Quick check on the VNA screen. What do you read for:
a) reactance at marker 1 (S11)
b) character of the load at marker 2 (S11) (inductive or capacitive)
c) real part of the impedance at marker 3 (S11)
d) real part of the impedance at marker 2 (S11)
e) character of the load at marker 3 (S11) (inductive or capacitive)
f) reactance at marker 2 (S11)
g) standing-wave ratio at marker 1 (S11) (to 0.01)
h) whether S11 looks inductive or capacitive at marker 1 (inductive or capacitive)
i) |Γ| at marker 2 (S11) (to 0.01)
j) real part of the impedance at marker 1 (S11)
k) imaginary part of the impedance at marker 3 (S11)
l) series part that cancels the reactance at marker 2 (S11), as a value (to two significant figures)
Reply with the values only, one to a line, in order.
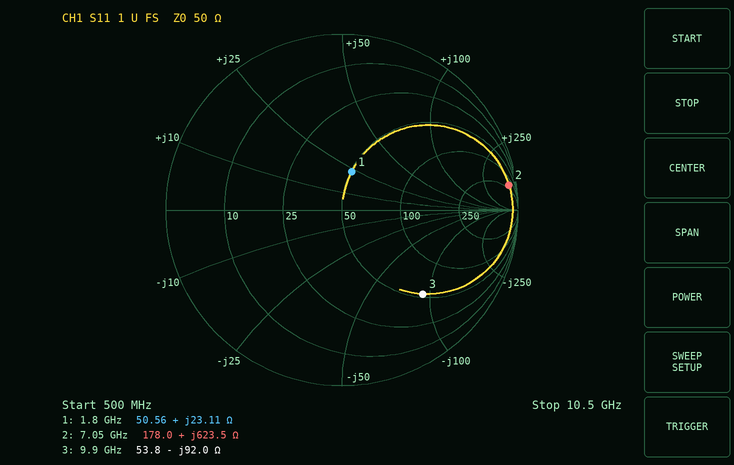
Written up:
+23.11 Ω
inductive
53.8 Ω
178.0 Ω
capacitive
+623.5 Ω
1.58
inductive
0.96
50.56 Ω
-92.0 Ω
36 fF
